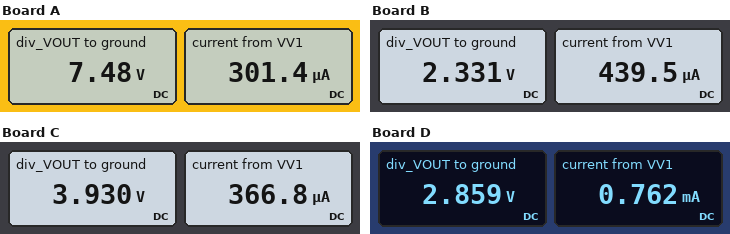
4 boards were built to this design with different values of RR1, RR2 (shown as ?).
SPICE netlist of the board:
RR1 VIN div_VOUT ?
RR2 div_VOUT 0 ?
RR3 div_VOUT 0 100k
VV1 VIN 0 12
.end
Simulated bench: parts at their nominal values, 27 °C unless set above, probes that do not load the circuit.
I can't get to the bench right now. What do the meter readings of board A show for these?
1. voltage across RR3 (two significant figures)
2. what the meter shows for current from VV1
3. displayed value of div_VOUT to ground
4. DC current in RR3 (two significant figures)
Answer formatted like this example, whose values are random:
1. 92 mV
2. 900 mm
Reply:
1. 7.5 V
2. 301.4 µA
3. 7.48 V
4. 75 µA
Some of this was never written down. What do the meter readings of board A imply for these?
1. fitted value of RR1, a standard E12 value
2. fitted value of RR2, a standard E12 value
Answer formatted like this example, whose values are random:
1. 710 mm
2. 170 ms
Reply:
1. 15 kΩ
2. 33 kΩ
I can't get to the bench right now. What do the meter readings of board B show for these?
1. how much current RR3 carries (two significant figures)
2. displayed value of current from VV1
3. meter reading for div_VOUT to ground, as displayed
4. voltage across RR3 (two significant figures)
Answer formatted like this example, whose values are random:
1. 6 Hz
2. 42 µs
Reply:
1. 23 µA
2. 439.5 µA
3. 2.331 V
4. 2.3 V
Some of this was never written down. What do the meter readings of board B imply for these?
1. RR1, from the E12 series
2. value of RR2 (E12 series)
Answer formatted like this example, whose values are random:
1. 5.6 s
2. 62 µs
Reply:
1. 22 kΩ
2. 5.6 kΩ
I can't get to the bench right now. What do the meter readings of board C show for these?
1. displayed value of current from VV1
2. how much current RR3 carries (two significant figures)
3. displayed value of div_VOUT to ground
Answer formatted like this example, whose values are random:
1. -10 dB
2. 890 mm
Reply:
1. 366.8 µA
2. 39 µA
3. 3.930 V
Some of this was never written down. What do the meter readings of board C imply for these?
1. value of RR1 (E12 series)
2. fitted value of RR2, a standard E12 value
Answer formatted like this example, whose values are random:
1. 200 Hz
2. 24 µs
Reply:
1. 22 kΩ
2. 12 kΩ
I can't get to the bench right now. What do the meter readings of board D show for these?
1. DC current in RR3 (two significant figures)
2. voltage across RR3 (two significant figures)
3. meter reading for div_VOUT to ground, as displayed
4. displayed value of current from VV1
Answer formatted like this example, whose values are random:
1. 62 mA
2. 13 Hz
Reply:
1. 29 µA
2. 2.9 V
3. 2.859 V
4. 0.762 mA
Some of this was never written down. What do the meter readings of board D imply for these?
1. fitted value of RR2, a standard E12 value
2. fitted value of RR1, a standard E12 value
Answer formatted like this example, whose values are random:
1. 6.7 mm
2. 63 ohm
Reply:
1. 3.9 kΩ
2. 12 kΩ
